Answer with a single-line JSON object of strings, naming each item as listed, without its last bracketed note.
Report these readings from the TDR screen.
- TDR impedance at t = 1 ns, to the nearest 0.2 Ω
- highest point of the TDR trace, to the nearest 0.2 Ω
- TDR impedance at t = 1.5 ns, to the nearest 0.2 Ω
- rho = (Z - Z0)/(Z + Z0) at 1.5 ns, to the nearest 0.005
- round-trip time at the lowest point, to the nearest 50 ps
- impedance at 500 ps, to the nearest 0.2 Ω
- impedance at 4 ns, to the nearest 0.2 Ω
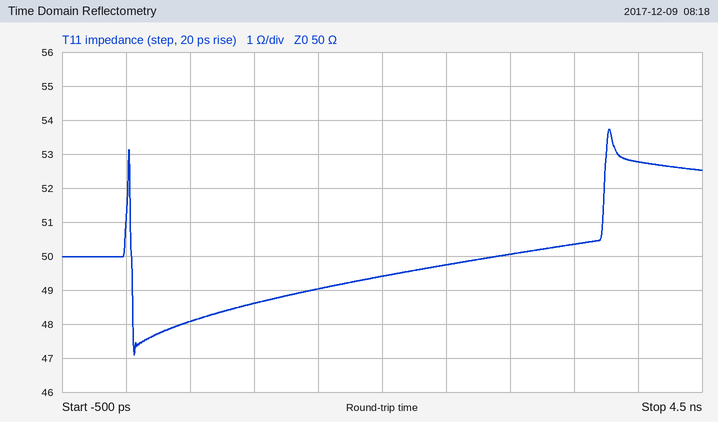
{"TDR impedance at t = 1 ns, to the nearest 0.2 Ω": "48.6 Ω", "highest point of the TDR trace, to the nearest 0.2 Ω": "53.8 Ω", "TDR impedance at t = 1.5 ns, to the nearest 0.2 Ω": "49.0 Ω", "rho = (Z - Z0)/(Z + Z0) at 1.5 ns, to the nearest 0.005": "-0.010", "round-trip time at the lowest point, to the nearest 50 ps": "50 ps", "impedance at 500 ps, to the nearest 0.2 Ω": "48.0 Ω", "impedance at 4 ns, to the nearest 0.2 Ω": "52.8 Ω"}
